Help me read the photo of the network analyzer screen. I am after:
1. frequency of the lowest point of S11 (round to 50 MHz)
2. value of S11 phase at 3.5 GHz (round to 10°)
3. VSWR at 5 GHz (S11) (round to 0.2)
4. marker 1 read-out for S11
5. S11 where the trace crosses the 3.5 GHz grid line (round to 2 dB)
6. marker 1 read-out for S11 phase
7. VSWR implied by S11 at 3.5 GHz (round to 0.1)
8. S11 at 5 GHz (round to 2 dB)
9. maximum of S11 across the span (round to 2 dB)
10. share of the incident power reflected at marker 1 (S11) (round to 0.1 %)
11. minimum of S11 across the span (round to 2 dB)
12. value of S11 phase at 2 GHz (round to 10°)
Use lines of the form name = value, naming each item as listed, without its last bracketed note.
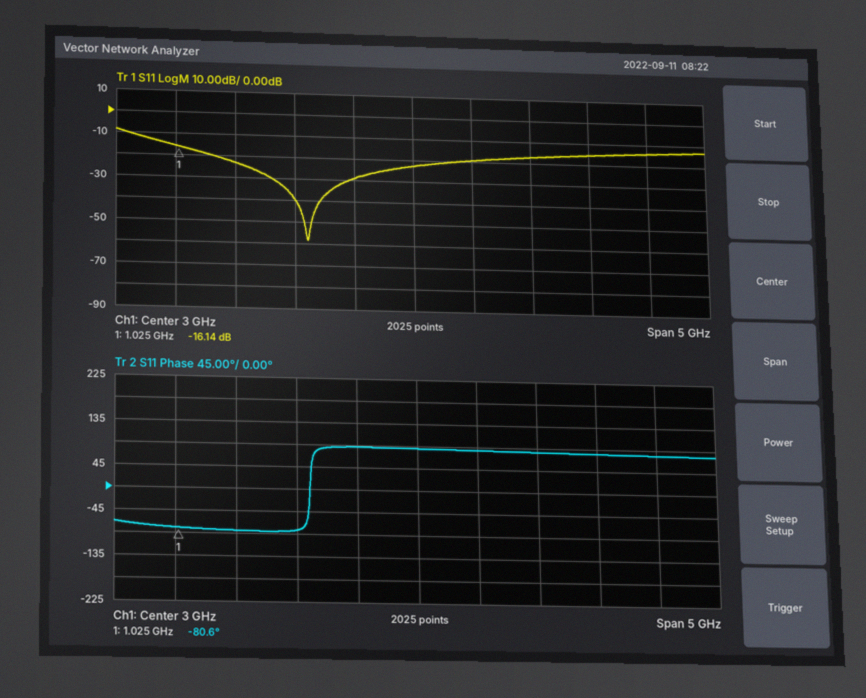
frequency of the lowest point of S11 = 2.10 GHz
value of S11 phase at 3.5 GHz = 80°
VSWR at 5 GHz (S11) = 1.4
marker 1 read-out for S11 = -16.14 dB
S11 where the trace crosses the 3.5 GHz grid line = -20 dB
marker 1 read-out for S11 phase = -80.6°
VSWR implied by S11 at 3.5 GHz = 1.2
S11 at 5 GHz = -14 dB
maximum of S11 across the span = -8 dB
share of the incident power reflected at marker 1 (S11) = 2.4 %
minimum of S11 across the span = -58 dB
value of S11 phase at 2 GHz = -80°
